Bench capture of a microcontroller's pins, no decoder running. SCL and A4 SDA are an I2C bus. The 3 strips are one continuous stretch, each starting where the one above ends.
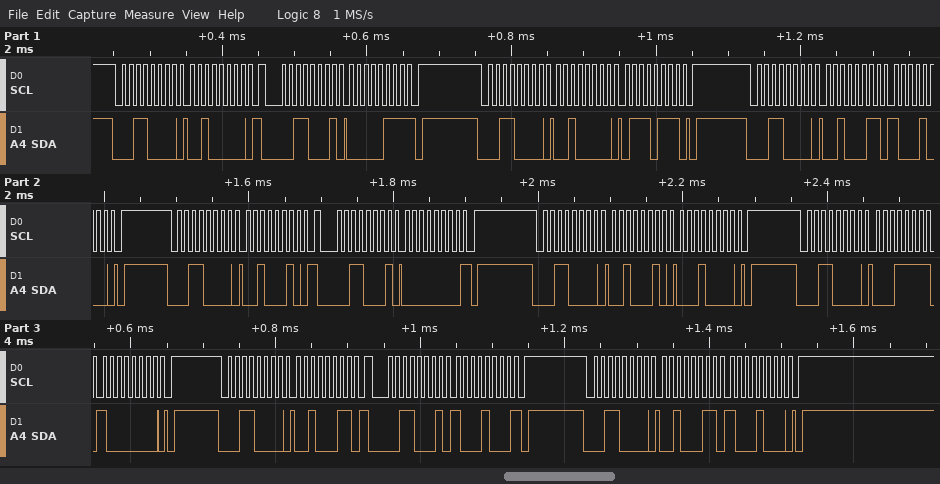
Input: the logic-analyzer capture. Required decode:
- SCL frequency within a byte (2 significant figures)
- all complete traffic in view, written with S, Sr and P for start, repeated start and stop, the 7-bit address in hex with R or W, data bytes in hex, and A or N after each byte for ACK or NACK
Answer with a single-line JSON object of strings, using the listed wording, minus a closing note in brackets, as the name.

{"SCL frequency within a byte": "100 kHz", "all complete traffic in view, written with S, Sr and P for start, repeated start and stop, the 7-bit address in hex with R or W, data bytes in hex, and A or N after each byte for ACK or NACK": "S 18W A 20 A Sr 18R A 07 N P S 18W A 20 A 77 A P S 18W A 23 A 88 A P S 18W A 22 A Sr 18R A 00 N P S 18W A 22 A 10 A P S 18W A 1F A 80 A P S 18W A 23 A Sr 18R A 88 N P S 18W A 23 A 88 A P"}
